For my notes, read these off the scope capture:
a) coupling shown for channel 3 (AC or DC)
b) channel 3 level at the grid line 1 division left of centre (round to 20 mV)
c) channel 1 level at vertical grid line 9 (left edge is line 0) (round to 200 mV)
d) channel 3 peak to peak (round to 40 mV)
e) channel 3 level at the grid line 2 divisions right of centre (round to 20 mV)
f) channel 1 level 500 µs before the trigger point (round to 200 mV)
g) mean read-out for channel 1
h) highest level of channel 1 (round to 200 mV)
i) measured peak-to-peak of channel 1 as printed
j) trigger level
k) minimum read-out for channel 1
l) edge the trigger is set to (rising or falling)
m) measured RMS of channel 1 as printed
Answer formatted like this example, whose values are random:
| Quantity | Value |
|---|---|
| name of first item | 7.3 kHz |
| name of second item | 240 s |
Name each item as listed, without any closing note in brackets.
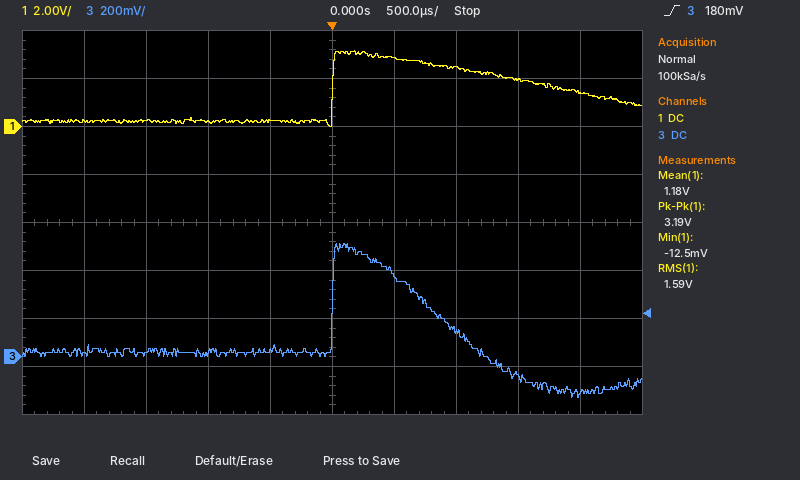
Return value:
| Quantity | Value |
|---|---|
| coupling shown for channel 3 | DC |
| channel 3 level at the grid line 1 division left of centre | 20 mV |
| channel 1 level at vertical grid line 9 (left edge is line 0) | 1.4 V |
| channel 3 peak to peak | 640 mV |
| channel 3 level at the grid line 2 divisions right of centre | 120 mV |
| channel 1 level 500 µs before the trigger point | 200 mV |
| mean read-out for channel 1 | 1.18 V |
| highest level of channel 1 | 3.2 V |
| measured peak-to-peak of channel 1 as printed | 3.19 V |
| trigger level | 180 mV |
| minimum read-out for channel 1 | -12.5 mV |
| edge the trigger is set to | rising |
| measured RMS of channel 1 as printed | 1.59 V |
